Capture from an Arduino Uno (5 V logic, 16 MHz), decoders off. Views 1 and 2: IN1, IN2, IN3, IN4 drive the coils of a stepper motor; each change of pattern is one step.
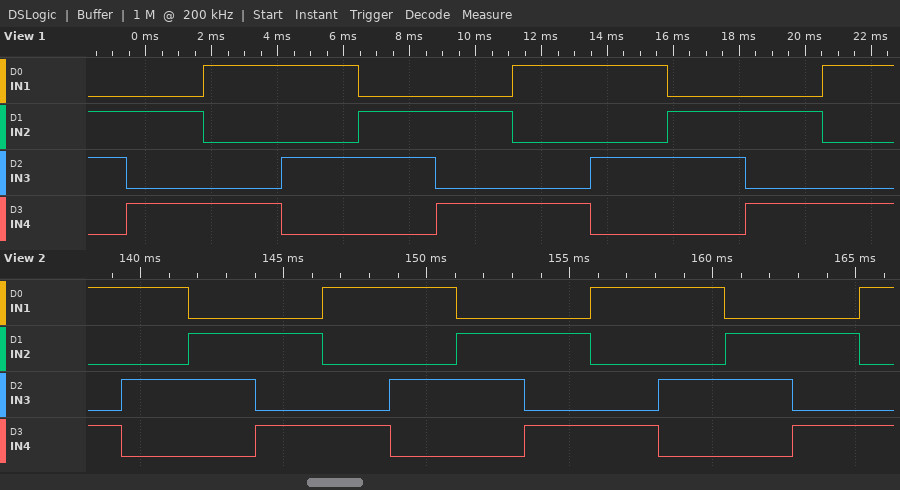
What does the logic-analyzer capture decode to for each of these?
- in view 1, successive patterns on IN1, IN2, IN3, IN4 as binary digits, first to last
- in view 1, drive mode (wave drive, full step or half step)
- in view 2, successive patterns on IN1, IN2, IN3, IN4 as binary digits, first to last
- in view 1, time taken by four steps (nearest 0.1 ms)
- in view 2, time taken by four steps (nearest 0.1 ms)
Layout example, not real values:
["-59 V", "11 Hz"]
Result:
["0110 0101 1001 1010 0110 0101 1001 1010 0110 0101 1001", "full step", "1001 1010 0110 0101 1001 1010 0110 0101 1001 1010 0110 0101 1001", "9.4 ms", "9.4 ms"]
